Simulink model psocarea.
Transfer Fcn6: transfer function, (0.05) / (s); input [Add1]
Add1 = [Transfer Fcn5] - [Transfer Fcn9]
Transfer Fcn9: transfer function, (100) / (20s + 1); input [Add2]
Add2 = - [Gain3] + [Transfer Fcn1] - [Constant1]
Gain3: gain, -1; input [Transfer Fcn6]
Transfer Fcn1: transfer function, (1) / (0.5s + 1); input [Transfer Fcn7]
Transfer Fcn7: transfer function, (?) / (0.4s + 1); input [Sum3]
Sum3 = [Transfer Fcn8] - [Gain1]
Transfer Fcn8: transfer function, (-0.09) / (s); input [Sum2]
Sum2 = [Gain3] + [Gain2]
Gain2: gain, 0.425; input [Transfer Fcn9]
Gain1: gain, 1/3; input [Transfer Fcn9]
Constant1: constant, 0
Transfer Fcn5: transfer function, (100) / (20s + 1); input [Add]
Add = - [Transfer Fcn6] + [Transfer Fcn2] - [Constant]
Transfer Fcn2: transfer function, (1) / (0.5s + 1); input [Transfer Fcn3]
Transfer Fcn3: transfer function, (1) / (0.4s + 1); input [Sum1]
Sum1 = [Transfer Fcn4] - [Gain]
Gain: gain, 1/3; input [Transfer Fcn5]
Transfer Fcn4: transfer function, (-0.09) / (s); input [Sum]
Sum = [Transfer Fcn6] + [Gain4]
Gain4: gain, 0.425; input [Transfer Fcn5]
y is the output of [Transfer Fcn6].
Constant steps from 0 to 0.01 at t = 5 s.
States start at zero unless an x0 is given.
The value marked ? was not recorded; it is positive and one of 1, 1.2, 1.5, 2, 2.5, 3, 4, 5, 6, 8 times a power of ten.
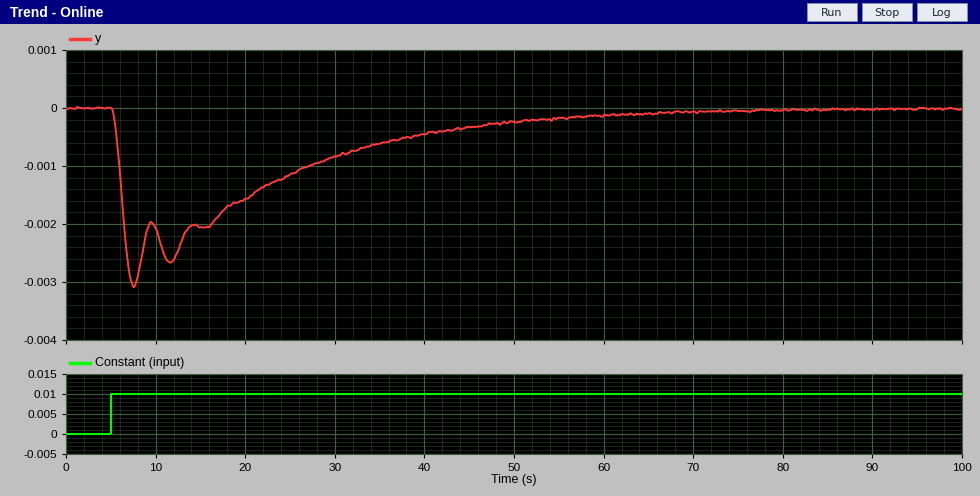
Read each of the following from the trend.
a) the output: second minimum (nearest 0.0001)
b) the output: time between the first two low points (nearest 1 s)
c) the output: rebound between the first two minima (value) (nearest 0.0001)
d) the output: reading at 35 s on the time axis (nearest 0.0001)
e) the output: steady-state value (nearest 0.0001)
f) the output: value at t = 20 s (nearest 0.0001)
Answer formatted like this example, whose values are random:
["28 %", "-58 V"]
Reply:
["-0.0027", "4 s", "-0.0020", "-0.0006", "0.0000", "-0.0016"]
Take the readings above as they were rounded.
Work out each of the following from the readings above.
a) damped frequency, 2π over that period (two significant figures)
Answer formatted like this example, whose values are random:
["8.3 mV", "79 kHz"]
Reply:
["1.6 rad/s"]
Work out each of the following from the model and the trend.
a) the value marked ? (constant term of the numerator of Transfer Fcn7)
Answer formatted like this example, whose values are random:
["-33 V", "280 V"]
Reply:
["0.6"]
